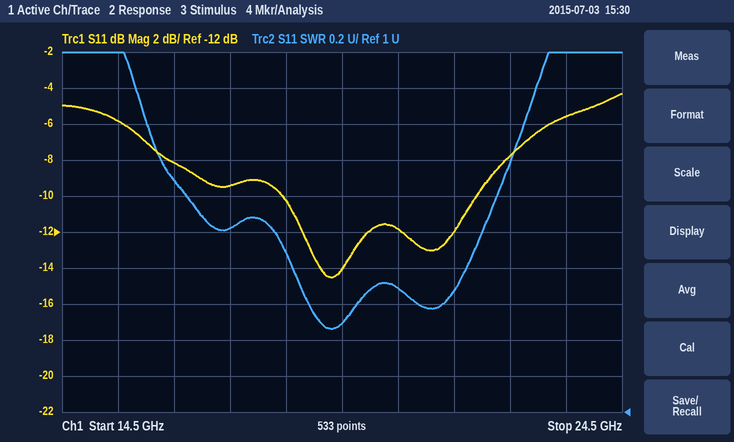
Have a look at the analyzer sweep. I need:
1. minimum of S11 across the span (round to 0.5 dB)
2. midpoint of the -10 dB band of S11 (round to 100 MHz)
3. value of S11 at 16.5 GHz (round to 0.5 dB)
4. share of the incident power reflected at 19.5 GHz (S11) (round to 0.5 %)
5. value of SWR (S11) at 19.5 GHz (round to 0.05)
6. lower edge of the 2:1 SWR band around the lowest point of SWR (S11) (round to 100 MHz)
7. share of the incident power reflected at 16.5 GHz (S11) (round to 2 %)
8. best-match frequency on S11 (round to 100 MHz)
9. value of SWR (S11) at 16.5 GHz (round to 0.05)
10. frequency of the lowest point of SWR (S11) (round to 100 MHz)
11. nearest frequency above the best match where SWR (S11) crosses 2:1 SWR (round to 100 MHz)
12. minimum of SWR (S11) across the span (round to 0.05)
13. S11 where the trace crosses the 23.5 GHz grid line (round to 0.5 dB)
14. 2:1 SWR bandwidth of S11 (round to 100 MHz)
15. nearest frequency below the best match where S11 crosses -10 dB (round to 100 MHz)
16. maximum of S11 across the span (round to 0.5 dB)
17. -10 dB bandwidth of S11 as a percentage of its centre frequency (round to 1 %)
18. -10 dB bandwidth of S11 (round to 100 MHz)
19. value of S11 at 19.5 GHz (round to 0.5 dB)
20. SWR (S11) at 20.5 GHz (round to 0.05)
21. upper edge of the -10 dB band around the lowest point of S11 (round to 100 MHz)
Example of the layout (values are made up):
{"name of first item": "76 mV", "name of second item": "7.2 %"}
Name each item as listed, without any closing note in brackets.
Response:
{"minimum of S11 across the span": "-14.5 dB", "midpoint of the -10 dB band of S11": "20.2 GHz", "value of S11 at 16.5 GHz": "-8.0 dB", "share of the incident power reflected at 19.5 GHz (S11)": "4.0 %", "value of SWR (S11) at 19.5 GHz": "1.50", "lower edge of the 2:1 SWR band around the lowest point of SWR (S11)": "18.3 GHz", "share of the incident power reflected at 16.5 GHz (S11)": "16 %", "best-match frequency on S11": "19.3 GHz", "value of SWR (S11) at 16.5 GHz": "2.30", "frequency of the lowest point of SWR (S11)": "19.3 GHz", "nearest frequency above the best match where SWR (S11) crosses 2:1 SWR": "22.0 GHz", "minimum of SWR (S11) across the span": "1.45", "S11 where the trace crosses the 23.5 GHz grid line": "-5.5 dB", "2:1 SWR bandwidth of S11": "3.7 GHz", "nearest frequency below the best match where S11 crosses -10 dB": "18.4 GHz", "maximum of S11 across the span": "-4.5 dB", "-10 dB bandwidth of S11 as a percentage of its centre frequency": "17 %", "-10 dB bandwidth of S11": "3.5 GHz", "value of S11 at 19.5 GHz": "-14.0 dB", "SWR (S11) at 20.5 GHz": "1.70", "upper edge of the -10 dB band around the lowest point of S11": "21.9 GHz"}
